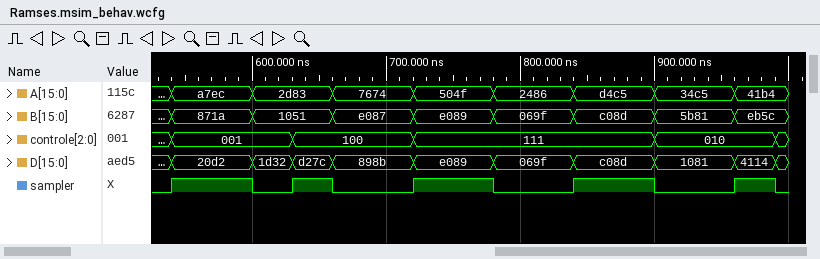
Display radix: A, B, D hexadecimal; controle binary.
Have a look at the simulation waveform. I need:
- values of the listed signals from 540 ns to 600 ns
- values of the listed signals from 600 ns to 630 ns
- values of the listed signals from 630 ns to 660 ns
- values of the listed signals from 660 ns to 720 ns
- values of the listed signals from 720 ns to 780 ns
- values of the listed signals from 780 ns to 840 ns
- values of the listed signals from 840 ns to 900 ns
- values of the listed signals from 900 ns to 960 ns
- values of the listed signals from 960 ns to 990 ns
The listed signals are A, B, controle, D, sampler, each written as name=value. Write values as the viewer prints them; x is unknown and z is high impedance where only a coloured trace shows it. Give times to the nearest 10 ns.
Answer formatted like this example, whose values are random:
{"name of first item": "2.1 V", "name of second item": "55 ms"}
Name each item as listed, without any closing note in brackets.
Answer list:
{"values of the listed signals from 540 ns to 600 ns": "A=a7ec, B=871a, controle=001, D=20d2, sampler=1", "values of the listed signals from 600 ns to 630 ns": "A=2d83, B=1051, controle=001, D=1d32, sampler=0", "values of the listed signals from 630 ns to 660 ns": "A=2d83, B=1051, controle=100, D=d27c, sampler=1", "values of the listed signals from 660 ns to 720 ns": "A=7674, B=e087, controle=100, D=898b, sampler=0", "values of the listed signals from 720 ns to 780 ns": "A=504f, B=e089, controle=111, D=e089, sampler=1", "values of the listed signals from 780 ns to 840 ns": "A=2486, B=069f, controle=111, D=069f, sampler=0", "values of the listed signals from 840 ns to 900 ns": "A=d4c5, B=c08d, controle=111, D=c08d, sampler=1", "values of the listed signals from 900 ns to 960 ns": "A=34c5, B=5b81, controle=010, D=1081, sampler=0", "values of the listed signals from 960 ns to 990 ns": "A=41b4, B=eb5c, controle=010, D=4114, sampler=1"}
